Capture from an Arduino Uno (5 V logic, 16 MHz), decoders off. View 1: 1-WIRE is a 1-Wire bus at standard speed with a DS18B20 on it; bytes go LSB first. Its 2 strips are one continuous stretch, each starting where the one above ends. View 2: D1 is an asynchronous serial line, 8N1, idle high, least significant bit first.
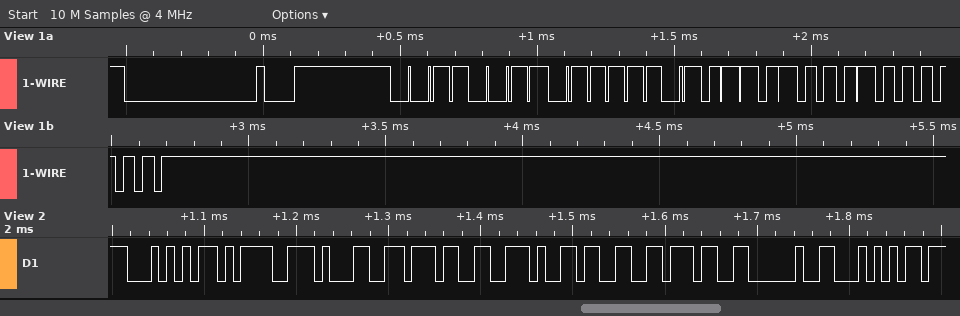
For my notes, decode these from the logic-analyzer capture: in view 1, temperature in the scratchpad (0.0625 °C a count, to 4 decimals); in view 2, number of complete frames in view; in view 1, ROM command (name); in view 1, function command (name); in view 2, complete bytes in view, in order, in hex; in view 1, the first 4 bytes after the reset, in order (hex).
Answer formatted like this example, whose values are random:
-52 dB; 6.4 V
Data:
17.3750 °C; 9; Skip ROM; Read Scratchpad; 54 3D 31 37 2E 33 37 20 54; CC BE 16 01
